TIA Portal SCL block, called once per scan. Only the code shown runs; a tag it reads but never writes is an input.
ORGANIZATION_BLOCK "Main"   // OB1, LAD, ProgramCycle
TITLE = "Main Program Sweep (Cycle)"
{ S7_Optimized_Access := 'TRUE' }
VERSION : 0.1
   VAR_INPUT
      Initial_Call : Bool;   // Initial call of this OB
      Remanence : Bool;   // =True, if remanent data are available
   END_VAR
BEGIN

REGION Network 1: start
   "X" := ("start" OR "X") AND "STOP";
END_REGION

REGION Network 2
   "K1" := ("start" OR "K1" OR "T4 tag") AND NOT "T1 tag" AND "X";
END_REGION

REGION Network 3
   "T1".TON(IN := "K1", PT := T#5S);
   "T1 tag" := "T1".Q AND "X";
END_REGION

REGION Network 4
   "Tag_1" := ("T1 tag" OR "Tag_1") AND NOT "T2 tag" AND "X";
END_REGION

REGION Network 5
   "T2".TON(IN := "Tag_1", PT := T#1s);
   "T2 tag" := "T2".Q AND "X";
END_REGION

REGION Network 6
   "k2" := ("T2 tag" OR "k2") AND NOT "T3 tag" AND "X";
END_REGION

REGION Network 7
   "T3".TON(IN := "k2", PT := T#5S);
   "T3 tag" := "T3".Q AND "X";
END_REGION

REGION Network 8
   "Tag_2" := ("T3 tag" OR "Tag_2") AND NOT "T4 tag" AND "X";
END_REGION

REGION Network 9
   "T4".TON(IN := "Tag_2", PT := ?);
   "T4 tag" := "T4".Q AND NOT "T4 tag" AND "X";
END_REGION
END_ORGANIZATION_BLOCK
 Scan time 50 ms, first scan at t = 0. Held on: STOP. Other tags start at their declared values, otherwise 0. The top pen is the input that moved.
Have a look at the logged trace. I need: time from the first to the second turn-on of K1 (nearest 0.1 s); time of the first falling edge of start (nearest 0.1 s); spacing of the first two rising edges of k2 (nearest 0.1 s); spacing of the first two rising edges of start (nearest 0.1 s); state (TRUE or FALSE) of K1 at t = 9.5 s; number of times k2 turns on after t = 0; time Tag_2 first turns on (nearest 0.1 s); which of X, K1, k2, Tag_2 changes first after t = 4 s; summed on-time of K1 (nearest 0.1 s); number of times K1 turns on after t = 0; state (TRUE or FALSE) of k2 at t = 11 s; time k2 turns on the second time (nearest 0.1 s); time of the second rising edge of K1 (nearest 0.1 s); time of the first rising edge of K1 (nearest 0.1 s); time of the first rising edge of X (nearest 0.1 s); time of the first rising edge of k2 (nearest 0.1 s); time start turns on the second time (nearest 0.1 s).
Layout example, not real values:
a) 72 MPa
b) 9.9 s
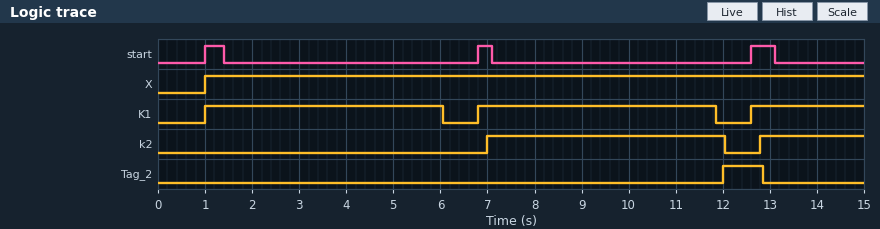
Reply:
a) 5.8 s
b) 1.4 s
c) 5.8 s
d) 5.8 s
e) TRUE
f) 2
g) 12.0 s
h) K1
i) 12.5 s
j) 3
k) TRUE
l) 12.8 s
m) 6.8 s
n) 1.0 s
o) 1.0 s
p) 7.0 s
q) 6.8 s
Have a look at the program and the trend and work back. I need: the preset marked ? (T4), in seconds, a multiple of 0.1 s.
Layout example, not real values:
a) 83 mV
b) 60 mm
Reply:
a) 0.8 s
